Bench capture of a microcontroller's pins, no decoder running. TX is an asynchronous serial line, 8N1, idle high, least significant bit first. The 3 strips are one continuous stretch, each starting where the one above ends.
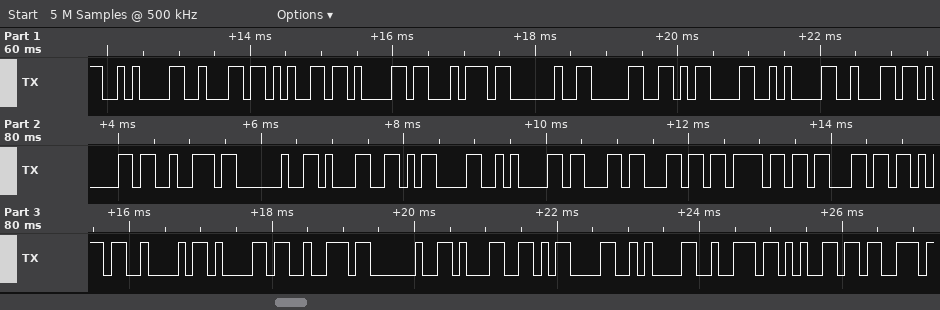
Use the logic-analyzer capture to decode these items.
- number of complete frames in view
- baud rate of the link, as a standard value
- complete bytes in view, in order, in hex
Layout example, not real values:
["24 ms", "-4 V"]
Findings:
["31", "9600 baud", "0A 62 65 61 74 20 30 0D 0A 62 61 72 20 31 0D 0A 63 6C 6F 63 6B 42 61 72 20 31 0D 0A 72 65 73"]
